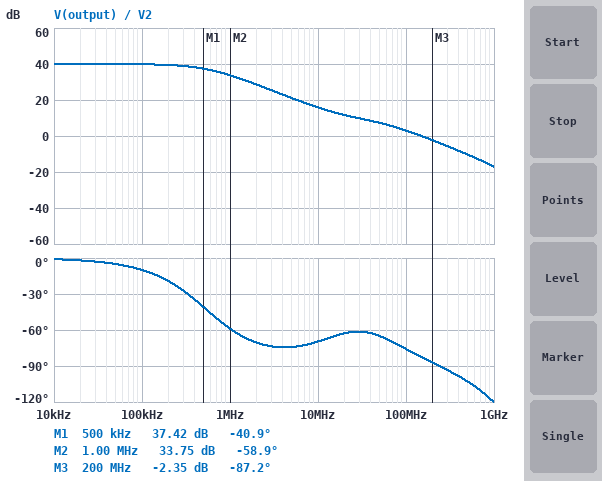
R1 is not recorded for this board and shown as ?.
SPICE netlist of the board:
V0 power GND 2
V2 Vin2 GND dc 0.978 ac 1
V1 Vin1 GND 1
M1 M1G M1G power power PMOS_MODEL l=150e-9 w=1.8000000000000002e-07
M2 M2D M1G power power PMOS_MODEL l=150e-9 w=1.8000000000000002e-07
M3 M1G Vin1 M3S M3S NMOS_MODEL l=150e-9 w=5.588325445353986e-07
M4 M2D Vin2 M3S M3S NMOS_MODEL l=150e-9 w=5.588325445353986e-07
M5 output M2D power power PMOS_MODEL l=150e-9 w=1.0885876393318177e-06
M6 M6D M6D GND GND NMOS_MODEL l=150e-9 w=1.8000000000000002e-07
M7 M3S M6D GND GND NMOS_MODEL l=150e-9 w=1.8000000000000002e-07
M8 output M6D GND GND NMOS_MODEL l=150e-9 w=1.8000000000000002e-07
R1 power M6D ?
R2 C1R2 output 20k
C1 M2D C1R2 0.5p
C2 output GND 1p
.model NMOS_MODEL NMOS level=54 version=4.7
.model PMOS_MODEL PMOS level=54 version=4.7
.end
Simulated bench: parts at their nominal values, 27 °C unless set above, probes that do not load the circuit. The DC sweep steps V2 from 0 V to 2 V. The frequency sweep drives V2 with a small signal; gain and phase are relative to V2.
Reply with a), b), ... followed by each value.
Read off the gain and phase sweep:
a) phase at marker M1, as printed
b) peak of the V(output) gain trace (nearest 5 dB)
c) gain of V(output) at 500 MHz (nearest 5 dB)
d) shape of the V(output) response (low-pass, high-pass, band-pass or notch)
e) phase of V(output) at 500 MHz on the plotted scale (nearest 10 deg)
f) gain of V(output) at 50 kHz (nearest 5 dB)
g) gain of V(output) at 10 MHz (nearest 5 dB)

a) -40.9 deg
b) 40 dB
c) -10 dB
d) low-pass
e) -100 deg
f) 40 dB
g) 15 dB
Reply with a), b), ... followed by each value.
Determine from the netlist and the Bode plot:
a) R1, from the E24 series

a) 16 kΩ
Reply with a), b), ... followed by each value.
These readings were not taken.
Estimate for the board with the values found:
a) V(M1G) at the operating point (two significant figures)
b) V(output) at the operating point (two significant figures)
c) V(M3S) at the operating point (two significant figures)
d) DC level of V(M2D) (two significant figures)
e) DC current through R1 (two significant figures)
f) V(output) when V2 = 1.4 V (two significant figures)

a) 1.1 V
b) 1.2 V
c) 480 mV
d) 1.4 V
e) 64 µA
f) 1.9 V
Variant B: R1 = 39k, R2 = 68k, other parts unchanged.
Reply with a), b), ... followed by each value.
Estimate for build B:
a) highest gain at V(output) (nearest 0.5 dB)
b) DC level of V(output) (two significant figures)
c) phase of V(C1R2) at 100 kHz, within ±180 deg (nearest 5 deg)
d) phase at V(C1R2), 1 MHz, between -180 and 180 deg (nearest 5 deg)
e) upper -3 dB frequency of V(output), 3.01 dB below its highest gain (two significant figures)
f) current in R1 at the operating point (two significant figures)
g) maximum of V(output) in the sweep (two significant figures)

a) 28.5 dB
b) 100 mV
c) -5 deg
d) -50 deg
e) 1.1 MHz
f) 32 µA
g) 2.0 V
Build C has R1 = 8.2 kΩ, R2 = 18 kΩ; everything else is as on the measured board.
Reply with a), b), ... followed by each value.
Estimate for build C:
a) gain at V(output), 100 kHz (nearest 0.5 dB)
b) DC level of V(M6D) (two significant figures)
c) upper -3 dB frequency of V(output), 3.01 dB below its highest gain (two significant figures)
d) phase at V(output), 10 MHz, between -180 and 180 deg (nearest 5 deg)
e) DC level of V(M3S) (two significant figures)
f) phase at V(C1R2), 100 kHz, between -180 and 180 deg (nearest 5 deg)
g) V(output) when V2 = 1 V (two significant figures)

a) 28.0 dB
b) 1.2 V
c) 1.8 MHz
d) -65 deg
e) 440 mV
f) -5 deg
g) 1.8 V
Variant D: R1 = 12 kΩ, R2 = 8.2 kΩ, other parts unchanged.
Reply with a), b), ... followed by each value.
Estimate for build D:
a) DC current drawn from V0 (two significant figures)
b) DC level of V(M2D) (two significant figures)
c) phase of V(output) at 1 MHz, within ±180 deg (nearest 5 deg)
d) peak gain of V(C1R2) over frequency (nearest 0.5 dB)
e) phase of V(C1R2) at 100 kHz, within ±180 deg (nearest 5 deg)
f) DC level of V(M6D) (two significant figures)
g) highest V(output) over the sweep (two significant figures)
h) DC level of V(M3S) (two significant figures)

a) 220 µA
b) 1.3 V
c) -50 deg
d) 36.0 dB
e) -5 deg
f) 1.1 V
g) 1.9 V
h) 460 mV
